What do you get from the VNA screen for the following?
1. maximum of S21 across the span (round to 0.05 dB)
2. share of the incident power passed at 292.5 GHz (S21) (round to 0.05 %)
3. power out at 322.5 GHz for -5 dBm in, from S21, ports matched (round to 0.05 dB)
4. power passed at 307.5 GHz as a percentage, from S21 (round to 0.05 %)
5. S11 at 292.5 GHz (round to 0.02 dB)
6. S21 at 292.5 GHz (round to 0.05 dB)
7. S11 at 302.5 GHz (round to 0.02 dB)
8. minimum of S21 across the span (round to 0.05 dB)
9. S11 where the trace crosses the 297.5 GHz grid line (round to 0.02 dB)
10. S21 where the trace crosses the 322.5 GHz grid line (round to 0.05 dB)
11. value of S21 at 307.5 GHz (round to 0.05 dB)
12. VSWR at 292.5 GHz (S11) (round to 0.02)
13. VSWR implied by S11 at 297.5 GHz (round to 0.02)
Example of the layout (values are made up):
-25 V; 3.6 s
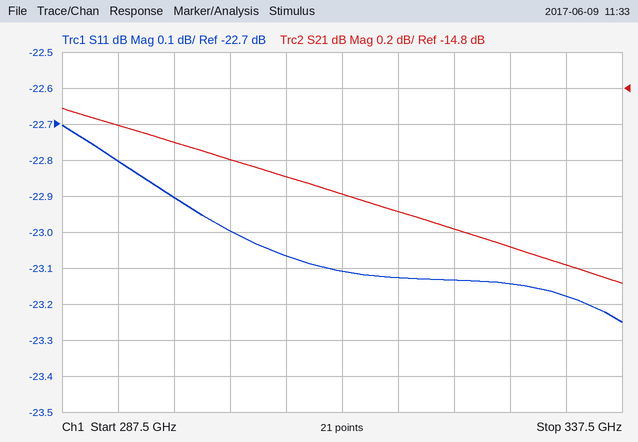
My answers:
-14.90 dB; 3.15 %; -20.60 dBm; 2.95 %; -22.80 dB; -15.00 dB; -23.00 dB; -15.90 dB; -22.90 dB; -15.60 dB; -15.30 dB; 1.16; 1.16
